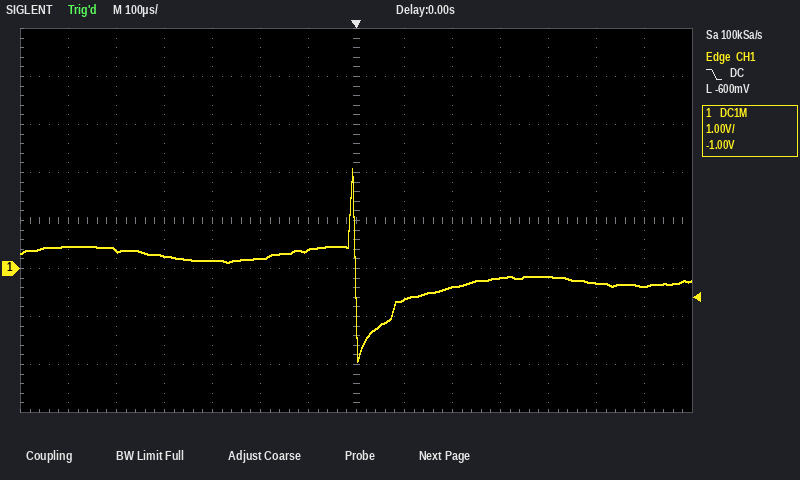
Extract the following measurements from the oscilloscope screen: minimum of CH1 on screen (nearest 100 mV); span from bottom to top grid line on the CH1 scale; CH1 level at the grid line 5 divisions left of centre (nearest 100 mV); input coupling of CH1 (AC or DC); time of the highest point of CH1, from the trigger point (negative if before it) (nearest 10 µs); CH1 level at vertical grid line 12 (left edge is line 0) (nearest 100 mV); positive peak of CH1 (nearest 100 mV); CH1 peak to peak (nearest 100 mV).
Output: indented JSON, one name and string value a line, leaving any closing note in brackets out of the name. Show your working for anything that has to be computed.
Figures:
{
  "minimum of CH1 on screen": "-1.9 V",
  "span from bottom to top grid line on the CH1 scale": "8 V",
  "CH1 level at the grid line 5 divisions left of centre": "400 mV",
  "input coupling of CH1": "DC",
  "time of the highest point of CH1, from the trigger point (negative if before it)": "-10 µs",
  "CH1 level at vertical grid line 12 (left edge is line 0)": "-300 mV",
  "positive peak of CH1": "2.1 V",
  "CH1 peak to peak": "2.1 V − (-1.9 V) = 4.0 V"
}
